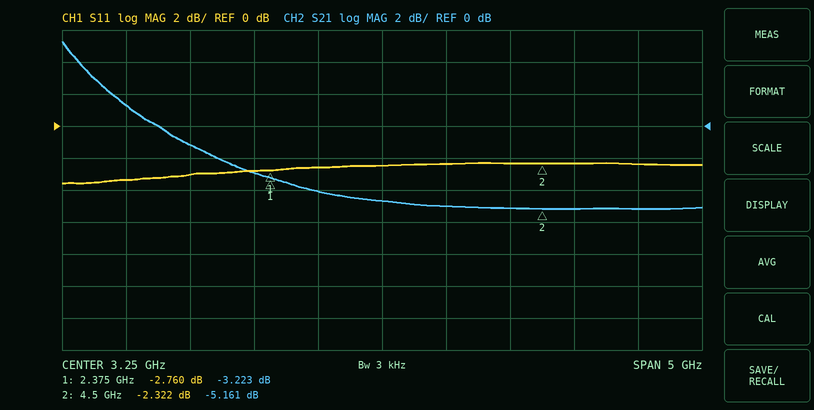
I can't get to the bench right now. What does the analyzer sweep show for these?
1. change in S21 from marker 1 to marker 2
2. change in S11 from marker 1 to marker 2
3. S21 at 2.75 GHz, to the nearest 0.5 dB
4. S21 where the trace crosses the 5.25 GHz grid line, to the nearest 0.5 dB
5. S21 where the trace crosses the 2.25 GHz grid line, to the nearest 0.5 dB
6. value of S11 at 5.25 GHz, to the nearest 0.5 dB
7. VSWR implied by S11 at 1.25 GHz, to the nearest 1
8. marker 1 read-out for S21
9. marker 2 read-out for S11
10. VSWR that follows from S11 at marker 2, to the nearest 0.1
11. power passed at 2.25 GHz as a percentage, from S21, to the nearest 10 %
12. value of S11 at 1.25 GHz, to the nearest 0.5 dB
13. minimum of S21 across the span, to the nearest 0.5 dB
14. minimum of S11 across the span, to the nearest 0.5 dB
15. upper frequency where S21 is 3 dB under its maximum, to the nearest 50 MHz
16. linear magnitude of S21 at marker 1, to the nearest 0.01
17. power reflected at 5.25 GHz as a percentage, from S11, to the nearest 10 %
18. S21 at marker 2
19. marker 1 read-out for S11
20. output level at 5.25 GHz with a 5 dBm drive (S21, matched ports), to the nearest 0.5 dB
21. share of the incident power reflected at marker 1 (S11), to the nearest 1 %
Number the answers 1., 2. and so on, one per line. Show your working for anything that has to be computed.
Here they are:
1. -5.161 − (-3.223) = -1.938 dB
2. -2.322 − (-2.76) = 0.438 dB
3. -4.0 dB
4. -5.0 dB
5. -3.0 dB
6. -2.5 dB
7. |Γ| = 10^(-3.5/20) = 0.6683; VSWR = (1 + 0.6683)/(1 − 0.6683) ≈ 5
8. -3.223 dB
9. -2.322 dB
10. (1 + 0.7654)/(1 − 0.7654) ≈ 7.5
11. 10^(-3/10) ≈ 50 %
12. -3.5 dB
13. -5.0 dB
14. -3.5 dB
15. 1.10 GHz
16. 10^(-3.223/20) ≈ 0.69
17. 10^(-2.5/10) ≈ 56.2 %, so 60 % to the nearest 10 %
18. -5.161 dB
19. -2.760 dB
20. 5 dBm + (-5.0 dB) = 0.0 dBm
21. 10^(-2.76/10) ≈ 53 %
